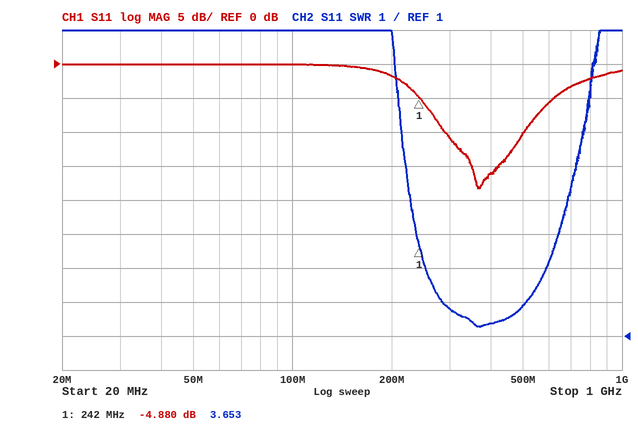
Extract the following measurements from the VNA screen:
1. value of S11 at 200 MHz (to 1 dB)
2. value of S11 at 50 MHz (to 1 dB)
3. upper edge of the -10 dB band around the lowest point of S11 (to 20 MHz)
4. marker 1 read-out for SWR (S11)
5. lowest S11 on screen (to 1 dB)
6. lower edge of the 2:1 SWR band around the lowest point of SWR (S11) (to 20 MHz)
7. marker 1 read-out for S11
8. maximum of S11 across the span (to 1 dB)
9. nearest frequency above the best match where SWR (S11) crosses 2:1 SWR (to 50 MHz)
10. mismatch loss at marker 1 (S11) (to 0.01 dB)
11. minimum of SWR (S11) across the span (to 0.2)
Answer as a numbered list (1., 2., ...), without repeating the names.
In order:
1. -2 dB
2. 0 dB
3. 500 MHz
4. 3.653
5. -18 dB
6. 280 MHz
7. -4.880 dB
8. 0 dB
9. 500 MHz
10. 1.71 dB
11. 1.2
